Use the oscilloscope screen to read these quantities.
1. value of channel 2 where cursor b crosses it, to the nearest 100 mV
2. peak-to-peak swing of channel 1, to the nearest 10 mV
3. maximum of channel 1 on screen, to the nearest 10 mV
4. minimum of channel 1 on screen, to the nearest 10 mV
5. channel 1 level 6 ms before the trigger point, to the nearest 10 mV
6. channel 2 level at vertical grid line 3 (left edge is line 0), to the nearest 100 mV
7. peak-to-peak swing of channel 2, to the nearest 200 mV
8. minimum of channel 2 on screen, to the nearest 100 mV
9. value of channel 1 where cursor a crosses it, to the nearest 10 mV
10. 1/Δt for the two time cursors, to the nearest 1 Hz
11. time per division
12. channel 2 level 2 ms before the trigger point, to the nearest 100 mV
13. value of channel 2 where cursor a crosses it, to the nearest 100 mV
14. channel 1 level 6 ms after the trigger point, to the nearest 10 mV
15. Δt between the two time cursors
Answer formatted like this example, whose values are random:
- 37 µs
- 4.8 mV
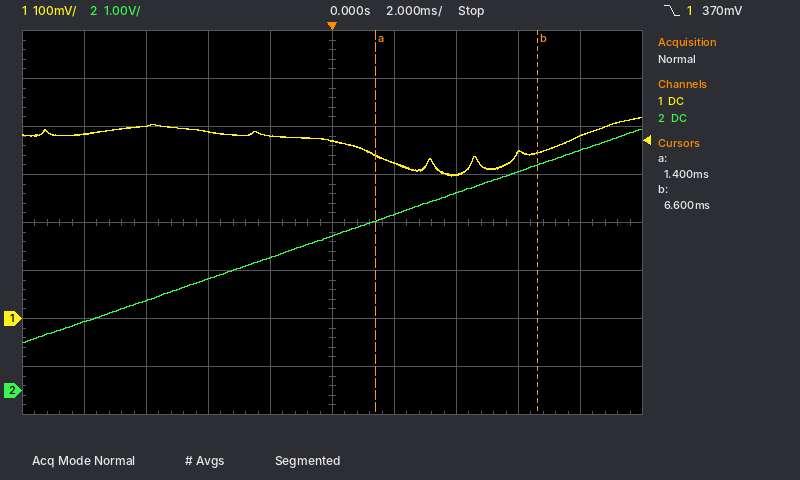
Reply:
- 4.7 V
- 120 mV
- 420 mV
- 300 mV
- 400 mV
- 2.3 V
- 4.4 V
- 1.0 V
- 340 mV
- 192 Hz
- 2 ms
- 2.8 V
- 3.5 V
- 340 mV
- 5.2 ms
